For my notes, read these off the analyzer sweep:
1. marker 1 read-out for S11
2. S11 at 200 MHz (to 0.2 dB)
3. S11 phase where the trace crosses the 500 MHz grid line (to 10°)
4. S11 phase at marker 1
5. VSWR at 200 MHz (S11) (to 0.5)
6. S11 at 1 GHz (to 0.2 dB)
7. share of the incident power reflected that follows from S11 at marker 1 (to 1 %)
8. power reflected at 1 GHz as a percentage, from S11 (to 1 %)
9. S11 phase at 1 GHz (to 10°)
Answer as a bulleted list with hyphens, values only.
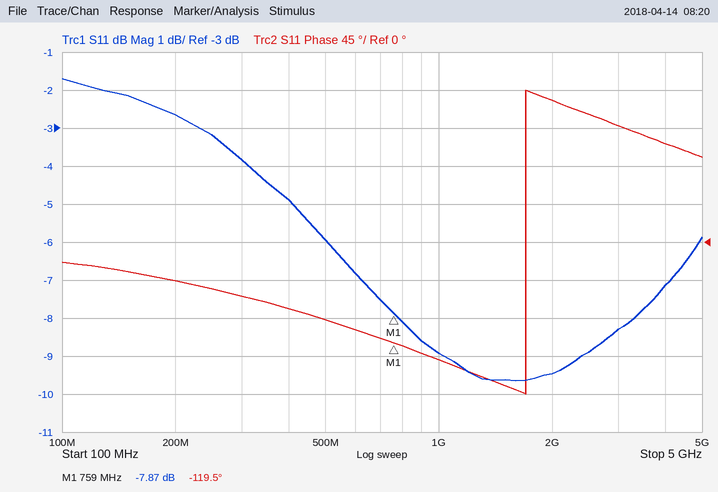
- -7.87 dB
- -2.6 dB
- -90°
- -119.5°
- 6.5
- -9.0 dB
- 16 %
- 13 %
- -140°
